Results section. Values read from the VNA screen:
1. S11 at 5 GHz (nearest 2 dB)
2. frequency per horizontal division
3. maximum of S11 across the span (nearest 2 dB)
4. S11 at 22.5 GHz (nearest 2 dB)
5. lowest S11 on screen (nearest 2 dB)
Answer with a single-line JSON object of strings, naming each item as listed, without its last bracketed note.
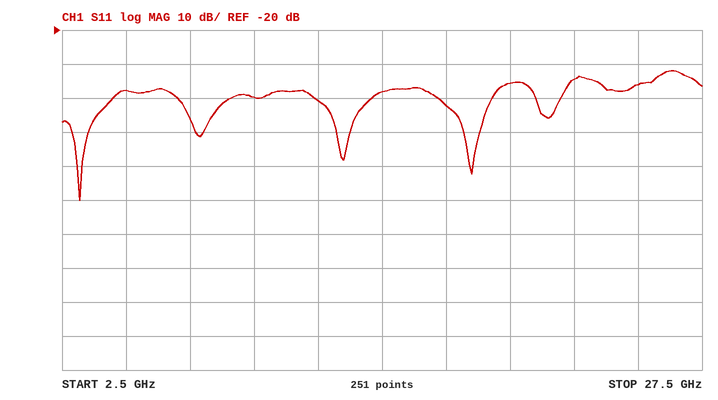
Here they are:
{"S11 at 5 GHz": "-38 dB", "frequency per horizontal division": "2.5 GHz", "maximum of S11 across the span": "-32 dB", "S11 at 22.5 GHz": "-34 dB", "lowest S11 on screen": "-70 dB"}
